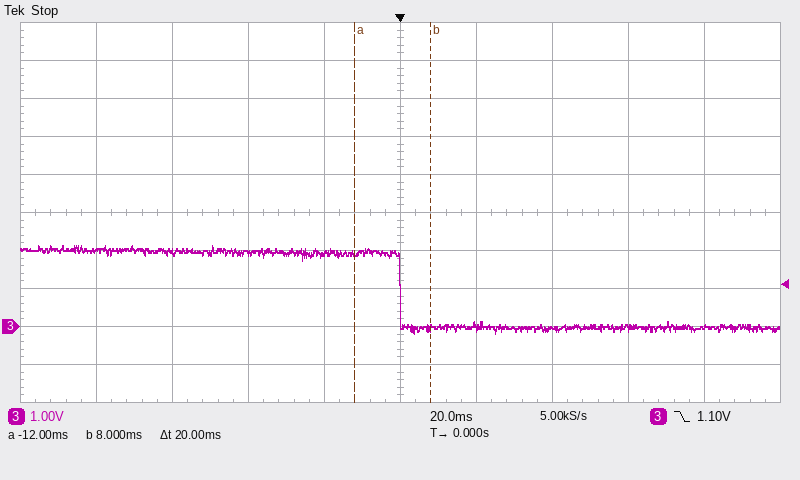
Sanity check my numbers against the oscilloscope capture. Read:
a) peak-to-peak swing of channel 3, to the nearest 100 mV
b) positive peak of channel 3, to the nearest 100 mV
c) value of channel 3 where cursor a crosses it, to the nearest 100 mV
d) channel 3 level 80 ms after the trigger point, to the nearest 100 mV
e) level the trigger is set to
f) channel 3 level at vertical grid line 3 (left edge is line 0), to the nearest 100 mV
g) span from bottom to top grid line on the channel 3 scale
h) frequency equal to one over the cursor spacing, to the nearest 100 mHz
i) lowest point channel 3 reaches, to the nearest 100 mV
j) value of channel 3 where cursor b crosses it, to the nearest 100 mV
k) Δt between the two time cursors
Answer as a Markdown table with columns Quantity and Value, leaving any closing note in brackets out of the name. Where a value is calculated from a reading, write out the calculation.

| Quantity | Value |
|---|---|
| peak-to-peak swing of channel 3, to the nearest 100 mV | 2.1 V − (-200 mV) = 2.3 V |
| positive peak of channel 3, to the nearest 100 mV | 2.1 V |
| value of channel 3 where cursor a crosses it, to the nearest 100 mV | 1.9 V |
| channel 3 level 80 ms after the trigger point, to the nearest 100 mV | 0.0 V |
| level the trigger is set to | 1.10 V |
| channel 3 level at vertical grid line 3 (left edge is line 0), to the nearest 100 mV | 1.9 V |
| span from bottom to top grid line on the channel 3 scale | 10 V |
| frequency equal to one over the cursor spacing, to the nearest 100 mHz | 1 / 20 ms ≈ 50.0 Hz |
| lowest point channel 3 reaches, to the nearest 100 mV | -200 mV |
| value of channel 3 where cursor b crosses it, to the nearest 100 mV | 0.0 V |
| Δt between the two time cursors | 20 ms |
